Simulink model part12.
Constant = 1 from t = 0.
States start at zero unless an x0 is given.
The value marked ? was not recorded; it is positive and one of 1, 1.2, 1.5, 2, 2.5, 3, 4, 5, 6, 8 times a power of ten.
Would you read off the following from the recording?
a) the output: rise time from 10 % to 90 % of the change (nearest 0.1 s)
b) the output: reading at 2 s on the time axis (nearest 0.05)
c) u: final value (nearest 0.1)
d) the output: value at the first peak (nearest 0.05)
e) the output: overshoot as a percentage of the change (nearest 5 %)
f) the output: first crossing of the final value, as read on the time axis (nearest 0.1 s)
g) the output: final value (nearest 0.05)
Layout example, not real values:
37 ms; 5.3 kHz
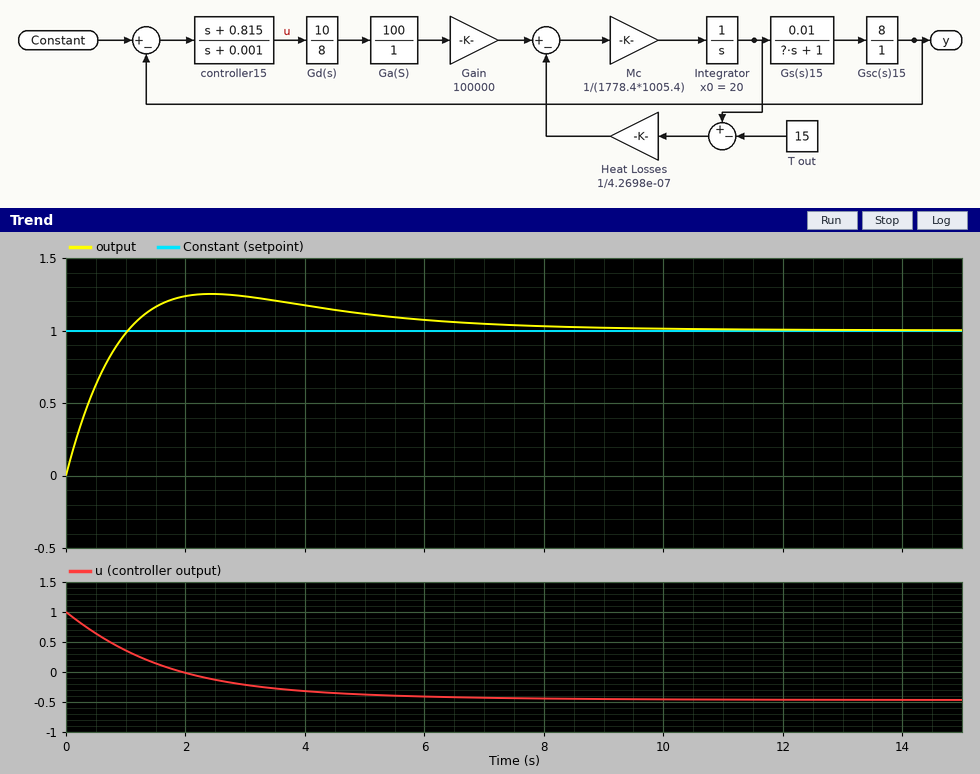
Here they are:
0.8 s; 1.25; -0.5; 1.25; 25 %; 1.0 s; 1.00
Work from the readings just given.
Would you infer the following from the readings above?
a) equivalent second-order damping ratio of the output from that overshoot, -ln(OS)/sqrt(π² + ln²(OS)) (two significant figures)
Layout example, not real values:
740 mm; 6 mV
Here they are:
0.40
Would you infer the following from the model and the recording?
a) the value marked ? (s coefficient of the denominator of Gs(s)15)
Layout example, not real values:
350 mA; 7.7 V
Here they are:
1
